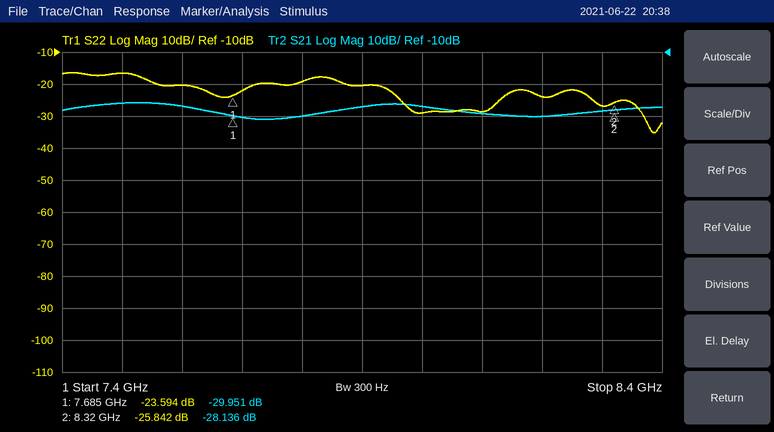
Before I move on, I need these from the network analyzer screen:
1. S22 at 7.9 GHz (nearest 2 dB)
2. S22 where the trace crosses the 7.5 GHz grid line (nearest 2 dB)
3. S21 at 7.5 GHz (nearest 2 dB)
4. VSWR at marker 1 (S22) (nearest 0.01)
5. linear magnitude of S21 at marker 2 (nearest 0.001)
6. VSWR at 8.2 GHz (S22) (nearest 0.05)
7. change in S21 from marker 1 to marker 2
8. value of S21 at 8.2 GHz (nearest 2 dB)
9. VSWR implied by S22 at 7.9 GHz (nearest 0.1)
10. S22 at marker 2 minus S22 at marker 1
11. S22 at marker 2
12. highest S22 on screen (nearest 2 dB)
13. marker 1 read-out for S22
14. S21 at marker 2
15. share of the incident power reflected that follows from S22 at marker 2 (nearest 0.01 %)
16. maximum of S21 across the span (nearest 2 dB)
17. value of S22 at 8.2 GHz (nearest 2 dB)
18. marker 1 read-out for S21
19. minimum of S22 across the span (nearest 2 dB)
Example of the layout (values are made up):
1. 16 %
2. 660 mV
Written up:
1. -20 dB
2. -16 dB
3. -26 dB
4. 1.14
5. 0.039
6. 1.15
7. 1.815 dB
8. -30 dB
9. 1.2
10. -2.248 dB
11. -25.842 dB
12. -16 dB
13. -23.594 dB
14. -28.136 dB
15. 0.26 %
16. -26 dB
17. -24 dB
18. -29.951 dB
19. -36 dB
